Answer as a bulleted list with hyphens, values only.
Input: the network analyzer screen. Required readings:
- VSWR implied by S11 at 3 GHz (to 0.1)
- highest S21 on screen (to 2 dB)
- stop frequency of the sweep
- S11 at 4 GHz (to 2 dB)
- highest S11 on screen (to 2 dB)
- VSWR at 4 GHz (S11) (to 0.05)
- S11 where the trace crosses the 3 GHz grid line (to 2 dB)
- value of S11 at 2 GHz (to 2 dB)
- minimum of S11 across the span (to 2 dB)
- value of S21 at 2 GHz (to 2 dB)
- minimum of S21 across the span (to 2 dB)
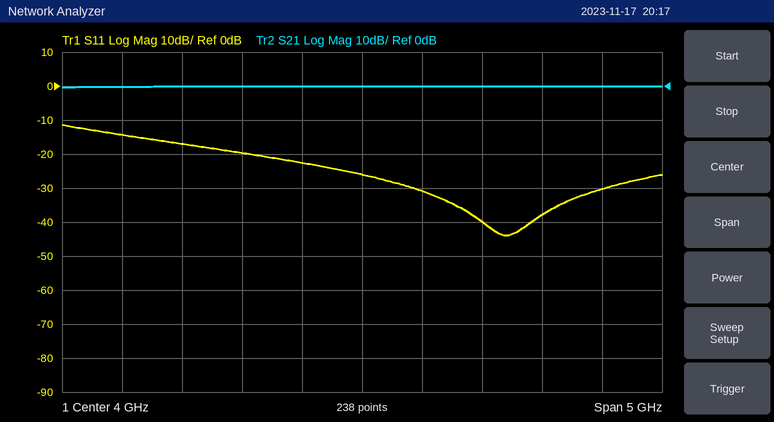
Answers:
- 1.2
- 0 dB
- 6.5 GHz
- -26 dB
- -12 dB
- 1.10
- -20 dB
- -14 dB
- -44 dB
- 0 dB
- 0 dB
